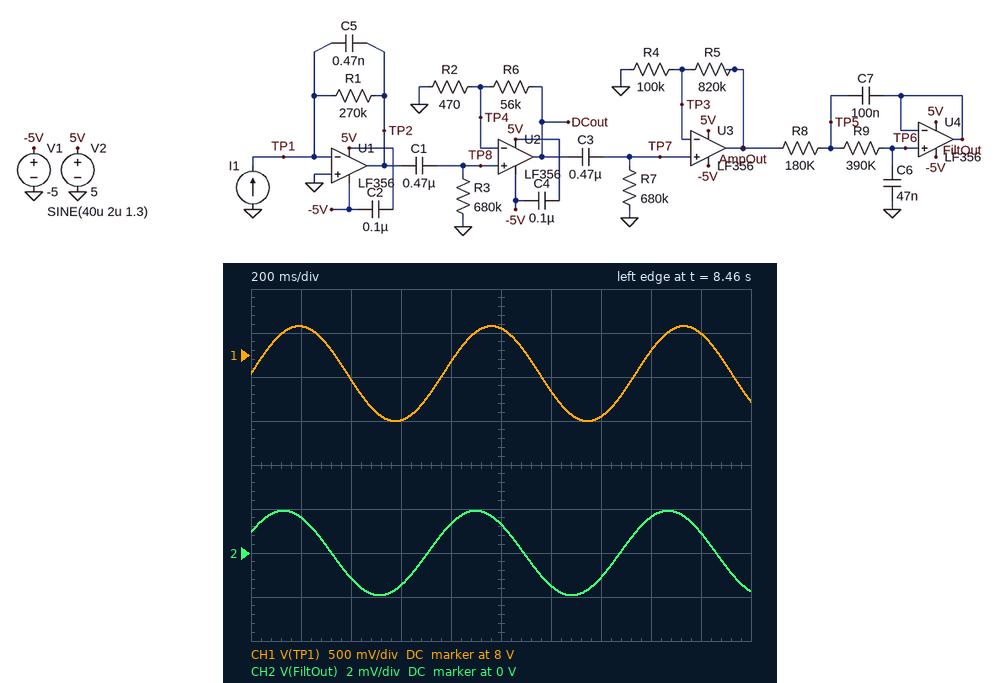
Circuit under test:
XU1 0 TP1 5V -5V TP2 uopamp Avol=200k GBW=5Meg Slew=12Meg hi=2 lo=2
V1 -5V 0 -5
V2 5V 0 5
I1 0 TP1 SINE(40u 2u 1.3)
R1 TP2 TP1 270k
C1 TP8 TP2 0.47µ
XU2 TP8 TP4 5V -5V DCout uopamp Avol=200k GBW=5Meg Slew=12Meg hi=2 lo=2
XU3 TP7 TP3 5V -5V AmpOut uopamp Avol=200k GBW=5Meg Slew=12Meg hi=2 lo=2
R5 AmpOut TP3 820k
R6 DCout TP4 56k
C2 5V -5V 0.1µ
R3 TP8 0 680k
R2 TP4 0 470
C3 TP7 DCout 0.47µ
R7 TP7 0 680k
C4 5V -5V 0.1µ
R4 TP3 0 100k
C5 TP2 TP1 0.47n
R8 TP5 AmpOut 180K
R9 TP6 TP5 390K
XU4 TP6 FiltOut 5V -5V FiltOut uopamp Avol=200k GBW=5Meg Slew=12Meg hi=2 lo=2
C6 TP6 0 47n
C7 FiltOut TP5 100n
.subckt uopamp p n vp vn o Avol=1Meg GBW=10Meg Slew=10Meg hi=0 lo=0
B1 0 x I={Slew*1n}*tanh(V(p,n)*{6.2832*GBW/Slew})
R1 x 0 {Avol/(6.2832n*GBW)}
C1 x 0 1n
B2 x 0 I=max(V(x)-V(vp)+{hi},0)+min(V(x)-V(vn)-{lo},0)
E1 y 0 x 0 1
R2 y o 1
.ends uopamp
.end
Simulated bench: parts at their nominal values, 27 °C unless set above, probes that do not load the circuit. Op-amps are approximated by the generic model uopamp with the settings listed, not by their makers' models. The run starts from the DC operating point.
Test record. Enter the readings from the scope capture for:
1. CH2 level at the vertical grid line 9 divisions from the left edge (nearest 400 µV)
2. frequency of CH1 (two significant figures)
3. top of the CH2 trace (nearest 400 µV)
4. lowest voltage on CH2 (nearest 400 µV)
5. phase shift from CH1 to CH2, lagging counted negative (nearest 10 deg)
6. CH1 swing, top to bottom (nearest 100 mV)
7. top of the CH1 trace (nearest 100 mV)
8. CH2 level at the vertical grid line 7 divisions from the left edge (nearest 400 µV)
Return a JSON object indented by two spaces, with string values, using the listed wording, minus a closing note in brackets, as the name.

{
  "CH2 level at the vertical grid line 9 divisions from the left edge": "800 µV",
  "frequency of CH1": "1.3 Hz",
  "top of the CH2 trace": "2.0 mV",
  "lowest voltage on CH2": "-2.0 mV",
  "phase shift from CH1 to CH2, lagging counted negative": "30 deg",
  "CH1 swing, top to bottom": "1.1 V",
  "top of the CH1 trace": "8.3 V",
  "CH2 level at the vertical grid line 7 divisions from the left edge": "-1.2 mV"
}
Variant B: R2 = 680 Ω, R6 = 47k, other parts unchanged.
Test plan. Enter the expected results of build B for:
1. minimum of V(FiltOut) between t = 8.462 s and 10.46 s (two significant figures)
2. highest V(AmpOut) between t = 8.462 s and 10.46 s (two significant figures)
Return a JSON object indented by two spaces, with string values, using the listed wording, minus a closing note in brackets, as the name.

{
  "minimum of V(FiltOut) between t = 8.462 s and 10.46 s": "-1.1 mV",
  "highest V(AmpOut) between t = 8.462 s and 10.46 s": "1.1 mV"
}
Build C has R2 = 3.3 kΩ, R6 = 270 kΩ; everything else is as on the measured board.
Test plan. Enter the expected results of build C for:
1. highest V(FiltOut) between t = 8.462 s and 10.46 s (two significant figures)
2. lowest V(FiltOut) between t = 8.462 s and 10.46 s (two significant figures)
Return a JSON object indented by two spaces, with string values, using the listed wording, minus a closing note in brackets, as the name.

{
  "highest V(FiltOut) between t = 8.462 s and 10.46 s": "1.3 mV",
  "lowest V(FiltOut) between t = 8.462 s and 10.46 s": "-1.3 mV"
}
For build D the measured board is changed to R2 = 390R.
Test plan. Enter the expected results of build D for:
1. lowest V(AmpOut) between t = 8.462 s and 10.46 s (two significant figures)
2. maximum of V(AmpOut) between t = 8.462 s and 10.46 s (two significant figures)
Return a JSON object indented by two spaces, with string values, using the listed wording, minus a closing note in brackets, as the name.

{
  "lowest V(AmpOut) between t = 8.462 s and 10.46 s": "-2.3 mV",
  "maximum of V(AmpOut) between t = 8.462 s and 10.46 s": "2.3 mV"
}
